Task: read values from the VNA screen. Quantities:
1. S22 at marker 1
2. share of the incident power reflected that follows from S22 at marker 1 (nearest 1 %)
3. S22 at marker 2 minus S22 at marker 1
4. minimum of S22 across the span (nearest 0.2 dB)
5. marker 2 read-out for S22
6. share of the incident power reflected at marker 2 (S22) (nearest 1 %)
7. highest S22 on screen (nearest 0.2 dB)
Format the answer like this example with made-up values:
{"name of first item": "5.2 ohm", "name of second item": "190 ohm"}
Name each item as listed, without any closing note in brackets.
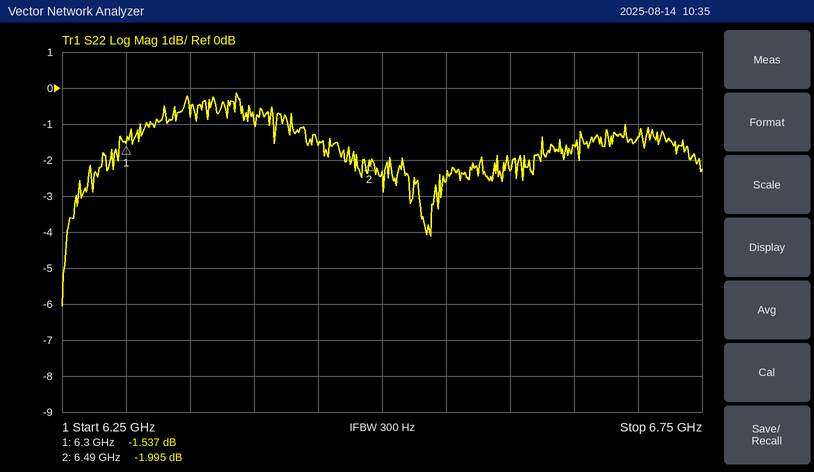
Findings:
{"S22 at marker 1": "-1.537 dB", "share of the incident power reflected that follows from S22 at marker 1": "70 %", "S22 at marker 2 minus S22 at marker 1": "-0.458 dB", "minimum of S22 across the span": "-6.0 dB", "marker 2 read-out for S22": "-1.995 dB", "share of the incident power reflected at marker 2 (S22)": "63 %", "highest S22 on screen": "-0.2 dB"}
